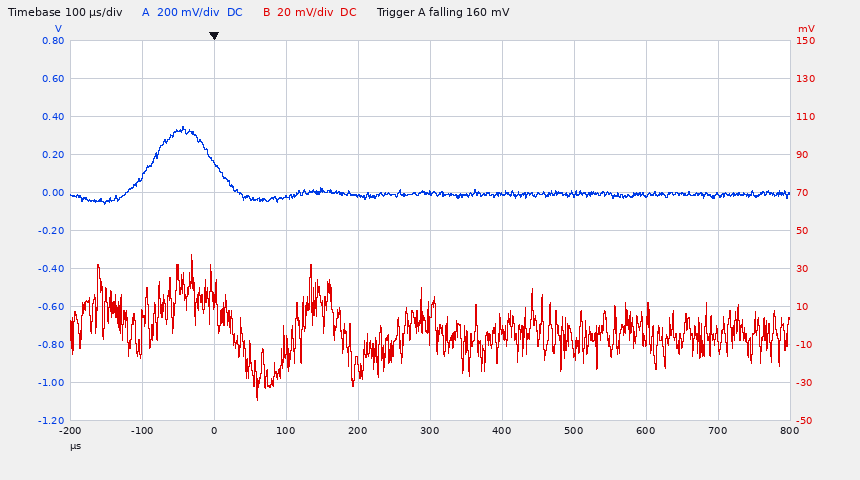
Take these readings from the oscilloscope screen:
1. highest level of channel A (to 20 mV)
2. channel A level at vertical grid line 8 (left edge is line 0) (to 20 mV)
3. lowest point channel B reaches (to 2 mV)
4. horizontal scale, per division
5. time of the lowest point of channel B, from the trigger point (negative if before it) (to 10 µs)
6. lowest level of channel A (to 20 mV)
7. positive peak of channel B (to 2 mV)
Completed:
340 mV
-20 mV
-40 mV
100 µs
+60 µs
-60 mV
38 mV
